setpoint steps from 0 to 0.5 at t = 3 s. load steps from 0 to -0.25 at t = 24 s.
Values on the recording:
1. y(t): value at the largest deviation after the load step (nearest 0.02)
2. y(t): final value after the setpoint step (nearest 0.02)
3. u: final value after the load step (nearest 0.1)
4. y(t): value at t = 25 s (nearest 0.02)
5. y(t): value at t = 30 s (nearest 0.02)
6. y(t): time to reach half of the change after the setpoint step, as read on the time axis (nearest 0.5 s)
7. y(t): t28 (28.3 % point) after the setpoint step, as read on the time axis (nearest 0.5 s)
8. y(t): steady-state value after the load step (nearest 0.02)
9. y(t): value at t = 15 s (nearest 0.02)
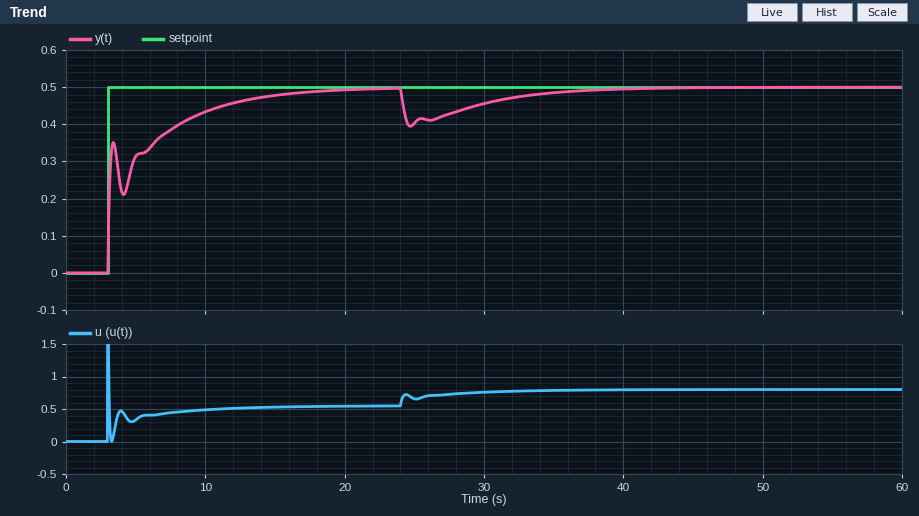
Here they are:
0.40
0.50
0.8
0.40
0.46
3.0 s
3.0 s
0.50
0.48
